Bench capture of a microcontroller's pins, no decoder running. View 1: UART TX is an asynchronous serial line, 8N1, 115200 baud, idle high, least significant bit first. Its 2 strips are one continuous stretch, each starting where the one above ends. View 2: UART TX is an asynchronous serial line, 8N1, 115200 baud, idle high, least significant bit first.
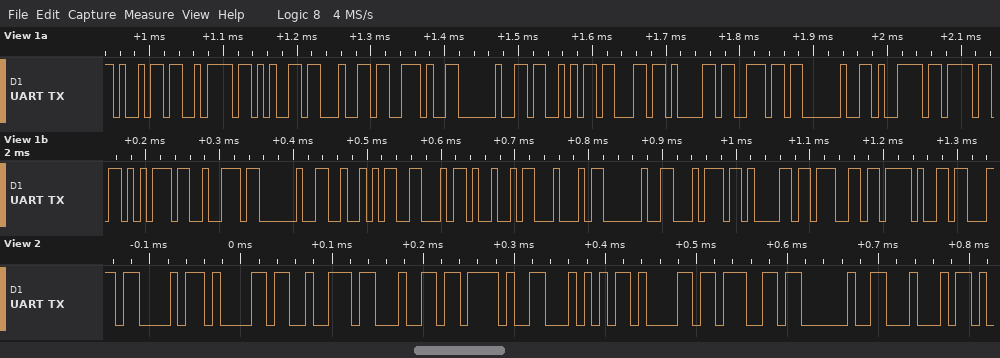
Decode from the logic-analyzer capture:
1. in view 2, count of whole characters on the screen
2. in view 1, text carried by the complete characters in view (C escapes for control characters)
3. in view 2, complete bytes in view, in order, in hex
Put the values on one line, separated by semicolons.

10; "ized. Scan your RFID tag/"; 43 61 72 64 2F 54 61 67 20 44
